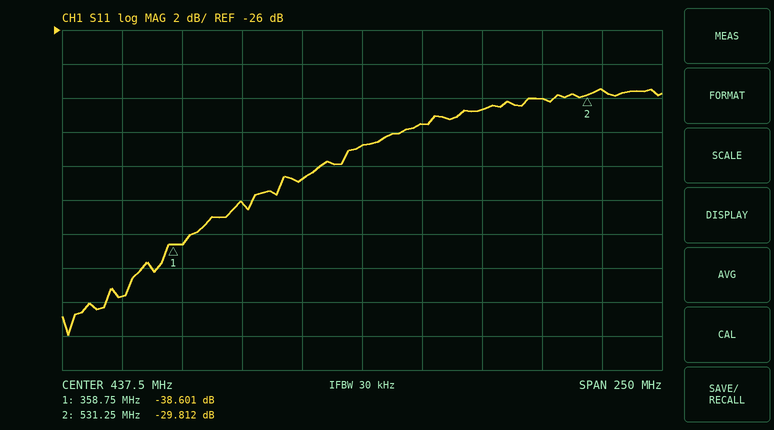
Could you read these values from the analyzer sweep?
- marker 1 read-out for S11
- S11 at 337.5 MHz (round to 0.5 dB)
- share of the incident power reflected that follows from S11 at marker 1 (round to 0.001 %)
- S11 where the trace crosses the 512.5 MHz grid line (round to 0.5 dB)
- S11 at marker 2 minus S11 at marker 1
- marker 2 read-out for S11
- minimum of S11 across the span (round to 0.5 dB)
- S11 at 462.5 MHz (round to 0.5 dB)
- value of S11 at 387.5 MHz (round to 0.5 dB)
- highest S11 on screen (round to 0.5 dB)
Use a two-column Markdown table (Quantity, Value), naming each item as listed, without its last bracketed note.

| Quantity | Value |
|---|---|
| marker 1 read-out for S11 | -38.601 dB |
| S11 at 337.5 MHz | -41.5 dB |
| share of the incident power reflected that follows from S11 at marker 1 | 0.014 % |
| S11 where the trace crosses the 512.5 MHz grid line | -30.0 dB |
| S11 at marker 2 minus S11 at marker 1 | 8.789 dB |
| marker 2 read-out for S11 | -29.812 dB |
| minimum of S11 across the span | -44.0 dB |
| S11 at 462.5 MHz | -31.5 dB |
| value of S11 at 387.5 MHz | -36.0 dB |
| highest S11 on screen | -29.5 dB |
